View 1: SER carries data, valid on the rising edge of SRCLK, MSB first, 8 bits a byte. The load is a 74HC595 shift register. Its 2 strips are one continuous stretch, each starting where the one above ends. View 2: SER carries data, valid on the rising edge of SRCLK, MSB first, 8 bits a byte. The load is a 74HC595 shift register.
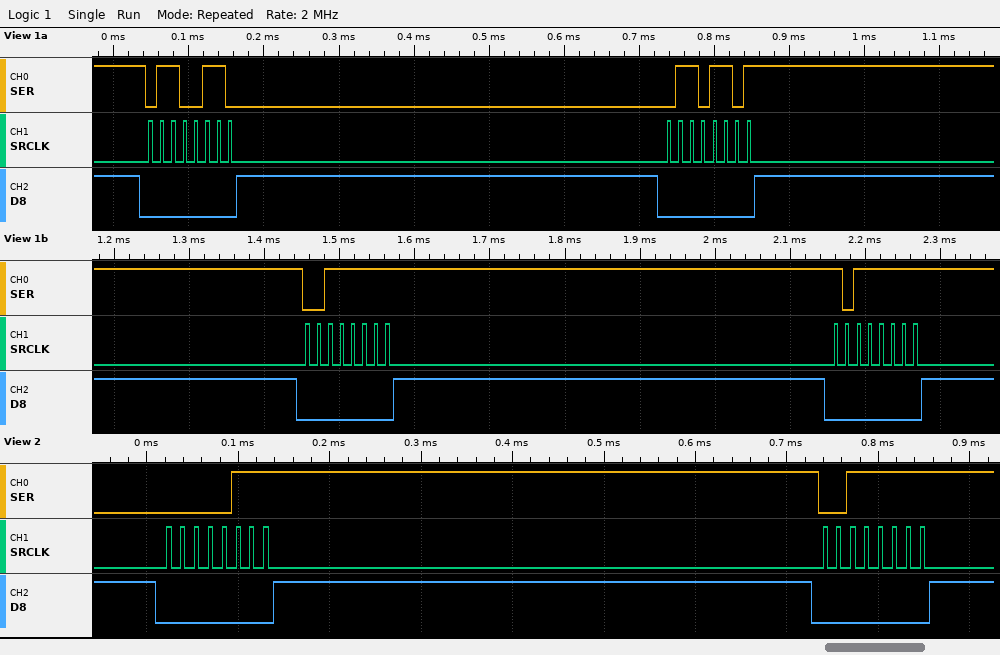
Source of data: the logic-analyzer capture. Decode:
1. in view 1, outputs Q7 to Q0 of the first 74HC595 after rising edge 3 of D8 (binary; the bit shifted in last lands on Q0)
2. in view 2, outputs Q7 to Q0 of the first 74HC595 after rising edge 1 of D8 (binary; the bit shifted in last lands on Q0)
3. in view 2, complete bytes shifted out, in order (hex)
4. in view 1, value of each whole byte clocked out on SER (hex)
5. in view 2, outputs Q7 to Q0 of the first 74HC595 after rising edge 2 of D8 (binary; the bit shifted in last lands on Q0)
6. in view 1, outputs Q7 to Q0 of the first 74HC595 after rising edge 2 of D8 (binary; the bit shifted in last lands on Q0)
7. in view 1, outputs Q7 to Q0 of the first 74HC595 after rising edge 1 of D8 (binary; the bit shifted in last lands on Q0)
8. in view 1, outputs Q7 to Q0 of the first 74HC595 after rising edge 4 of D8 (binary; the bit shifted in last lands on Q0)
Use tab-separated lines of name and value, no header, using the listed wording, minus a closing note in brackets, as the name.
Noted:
in view 1, outputs Q7 to Q0 of the first 74HC595 after rising edge 3 of D8	00111111
in view 2, outputs Q7 to Q0 of the first 74HC595 after rising edge 1 of D8	00000111
in view 2, complete bytes shifted out, in order	07 3F
in view 1, value of each whole byte clocked out on SER	0x66 0x6D 0x3F 0xBF
in view 2, outputs Q7 to Q0 of the first 74HC595 after rising edge 2 of D8	00111111
in view 1, outputs Q7 to Q0 of the first 74HC595 after rising edge 2 of D8	01101101
in view 1, outputs Q7 to Q0 of the first 74HC595 after rising edge 1 of D8	01100110
in view 1, outputs Q7 to Q0 of the first 74HC595 after rising edge 4 of D8	10111111
